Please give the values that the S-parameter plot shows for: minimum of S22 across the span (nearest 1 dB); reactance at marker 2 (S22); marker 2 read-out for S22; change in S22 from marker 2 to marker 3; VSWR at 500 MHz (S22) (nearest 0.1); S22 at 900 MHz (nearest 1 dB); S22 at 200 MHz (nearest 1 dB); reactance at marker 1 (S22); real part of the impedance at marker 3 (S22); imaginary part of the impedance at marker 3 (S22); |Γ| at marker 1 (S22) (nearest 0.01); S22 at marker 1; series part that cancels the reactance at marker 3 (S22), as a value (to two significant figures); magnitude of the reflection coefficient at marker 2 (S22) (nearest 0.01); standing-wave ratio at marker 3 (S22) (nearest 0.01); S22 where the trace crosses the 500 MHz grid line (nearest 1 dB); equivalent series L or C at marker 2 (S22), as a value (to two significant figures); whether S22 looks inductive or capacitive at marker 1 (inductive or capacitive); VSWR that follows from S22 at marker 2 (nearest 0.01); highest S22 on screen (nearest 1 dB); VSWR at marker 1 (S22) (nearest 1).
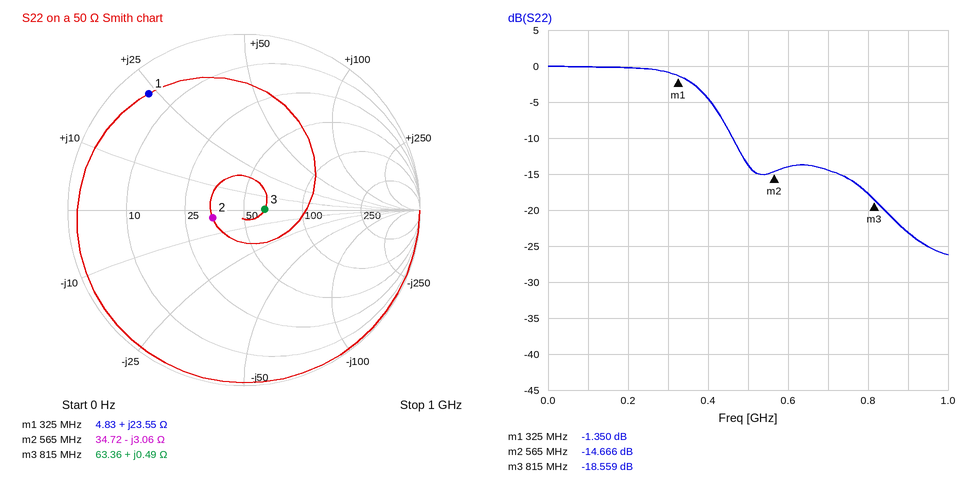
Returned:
-26 dB
-3.06 Ω
-14.666 dB
-3.893 dB
1.5
-23 dB
0 dB
+23.55 Ω
63.36 Ω
+0.49 Ω
0.85
-1.350 dB
400 pF
0.18
1.27
-14 dB
92 pF
inductive
1.45
0 dB
13
